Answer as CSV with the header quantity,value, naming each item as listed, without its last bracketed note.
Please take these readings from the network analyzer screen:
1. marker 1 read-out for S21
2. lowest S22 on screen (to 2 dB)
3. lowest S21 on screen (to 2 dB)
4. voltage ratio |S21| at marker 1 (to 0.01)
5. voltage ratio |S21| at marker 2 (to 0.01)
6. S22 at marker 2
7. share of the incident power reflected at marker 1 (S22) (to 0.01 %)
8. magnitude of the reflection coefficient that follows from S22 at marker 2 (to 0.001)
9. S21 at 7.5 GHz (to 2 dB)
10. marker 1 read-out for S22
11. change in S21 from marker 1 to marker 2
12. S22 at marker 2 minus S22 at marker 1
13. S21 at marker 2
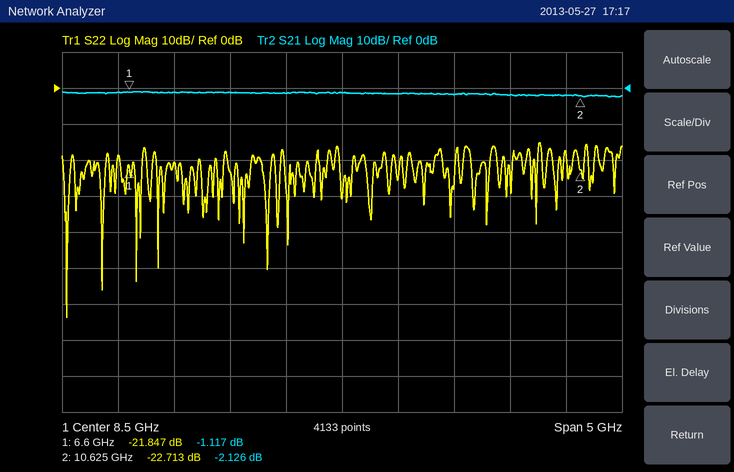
quantity,value
marker 1 read-out for S21,-1.117 dB
lowest S22 on screen,-64 dB
lowest S21 on screen,-2 dB
voltage ratio |S21| at marker 1,0.88
voltage ratio |S21| at marker 2,0.78
S22 at marker 2,-22.713 dB
share of the incident power reflected at marker 1 (S22),0.65 %
magnitude of the reflection coefficient that follows from S22 at marker 2,0.073
S21 at 7.5 GHz,-2 dB
marker 1 read-out for S22,-21.847 dB
change in S21 from marker 1 to marker 2,-1.009 dB
S22 at marker 2 minus S22 at marker 1,-0.866 dB
S21 at marker 2,-2.126 dB
